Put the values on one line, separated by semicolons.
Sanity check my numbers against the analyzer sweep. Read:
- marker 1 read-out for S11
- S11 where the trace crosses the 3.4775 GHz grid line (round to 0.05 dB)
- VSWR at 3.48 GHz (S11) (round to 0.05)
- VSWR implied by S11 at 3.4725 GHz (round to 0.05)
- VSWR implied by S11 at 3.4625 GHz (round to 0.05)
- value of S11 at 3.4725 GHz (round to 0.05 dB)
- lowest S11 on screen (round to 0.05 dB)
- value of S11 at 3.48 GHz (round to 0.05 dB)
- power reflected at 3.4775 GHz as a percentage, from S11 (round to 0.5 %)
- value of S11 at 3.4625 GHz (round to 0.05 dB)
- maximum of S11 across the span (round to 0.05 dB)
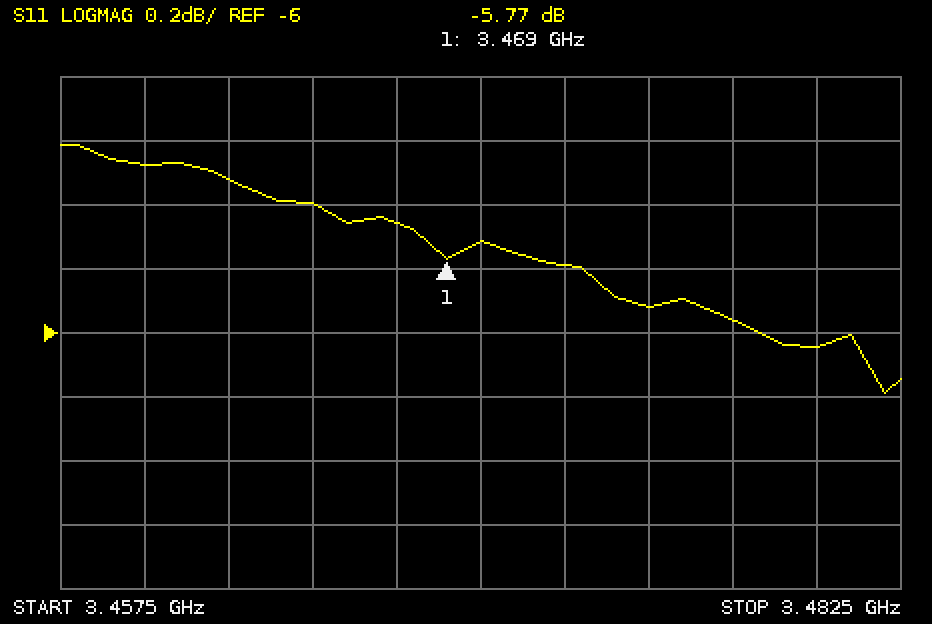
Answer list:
-5.77 dB; -5.95 dB; 3.00; 3.10; 3.25; -5.80 dB; -6.20 dB; -6.05 dB; 25.5 %; -5.50 dB; -5.40 dB
